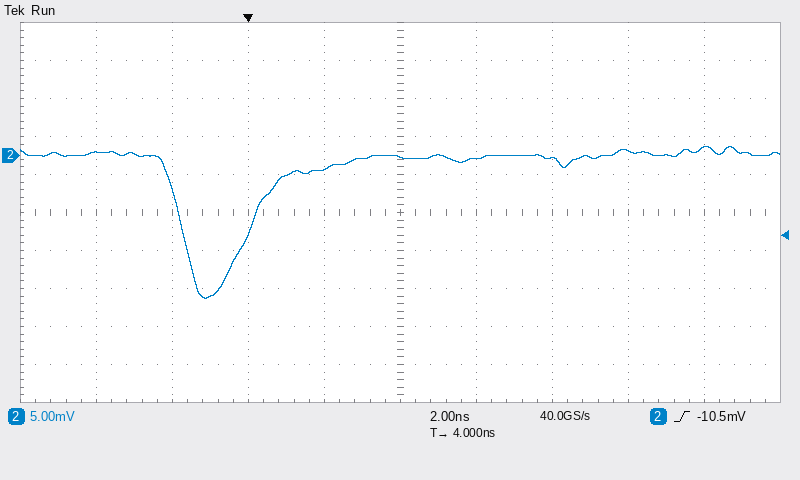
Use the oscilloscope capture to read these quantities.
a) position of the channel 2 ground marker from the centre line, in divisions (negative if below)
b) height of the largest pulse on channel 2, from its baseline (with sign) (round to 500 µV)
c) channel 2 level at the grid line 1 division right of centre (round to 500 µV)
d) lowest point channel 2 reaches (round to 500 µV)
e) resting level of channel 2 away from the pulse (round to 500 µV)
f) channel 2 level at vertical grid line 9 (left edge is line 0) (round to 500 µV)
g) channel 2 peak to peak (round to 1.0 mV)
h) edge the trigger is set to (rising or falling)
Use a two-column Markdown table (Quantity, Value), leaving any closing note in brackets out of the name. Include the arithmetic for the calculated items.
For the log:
| Quantity | Value |
|---|---|
| position of the channel 2 ground marker from the centre line, in divisions | +1.5 div |
| height of the largest pulse on channel 2, from its baseline (with sign) | -19.0 mV − (0.0 mV) = -19.0 mV |
| channel 2 level at the grid line 1 division right of centre | -500 µV |
| lowest point channel 2 reaches | -19.0 mV |
| resting level of channel 2 away from the pulse | 0.0 mV |
| channel 2 level at vertical grid line 9 (left edge is line 0) | 1.0 mV |
| channel 2 peak to peak | 20.0 mV |
| edge the trigger is set to | rising |
